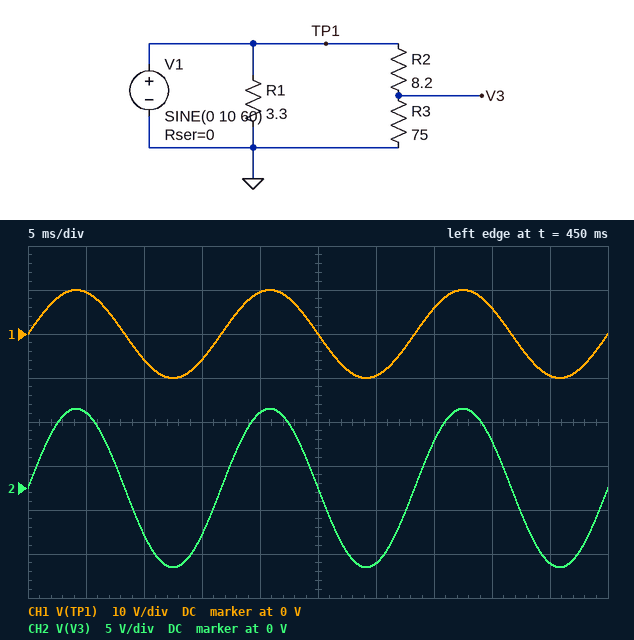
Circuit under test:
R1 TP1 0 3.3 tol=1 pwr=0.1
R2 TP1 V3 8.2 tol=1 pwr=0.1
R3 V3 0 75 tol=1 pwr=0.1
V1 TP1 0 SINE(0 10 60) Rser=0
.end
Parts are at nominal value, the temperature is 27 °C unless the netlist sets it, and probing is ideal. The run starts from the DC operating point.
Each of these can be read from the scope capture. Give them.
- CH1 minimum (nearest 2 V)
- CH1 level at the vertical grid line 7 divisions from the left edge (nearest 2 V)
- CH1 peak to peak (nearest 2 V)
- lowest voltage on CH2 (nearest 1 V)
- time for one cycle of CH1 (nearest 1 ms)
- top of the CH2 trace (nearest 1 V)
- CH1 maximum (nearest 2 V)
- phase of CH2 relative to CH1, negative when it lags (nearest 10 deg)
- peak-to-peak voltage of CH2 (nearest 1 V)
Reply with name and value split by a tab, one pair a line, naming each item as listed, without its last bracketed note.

CH1 minimum	-10 V
CH1 level at the vertical grid line 7 divisions from the left edge	6 V
CH1 peak to peak	20 V
lowest voltage on CH2	-9 V
time for one cycle of CH1	17 ms
top of the CH2 trace	9 V
CH1 maximum	10 V
phase of CH2 relative to CH1, negative when it lags	0 deg
peak-to-peak voltage of CH2	18 V
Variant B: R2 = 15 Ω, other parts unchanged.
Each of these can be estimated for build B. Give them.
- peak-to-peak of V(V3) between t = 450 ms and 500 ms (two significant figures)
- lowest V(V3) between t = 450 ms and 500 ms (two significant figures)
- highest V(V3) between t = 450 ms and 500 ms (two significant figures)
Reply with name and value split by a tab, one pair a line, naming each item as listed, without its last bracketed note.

peak-to-peak of V(V3) between t = 450 ms and 500 ms	17 V
lowest V(V3) between t = 450 ms and 500 ms	-8.3 V
highest V(V3) between t = 450 ms and 500 ms	8.3 V
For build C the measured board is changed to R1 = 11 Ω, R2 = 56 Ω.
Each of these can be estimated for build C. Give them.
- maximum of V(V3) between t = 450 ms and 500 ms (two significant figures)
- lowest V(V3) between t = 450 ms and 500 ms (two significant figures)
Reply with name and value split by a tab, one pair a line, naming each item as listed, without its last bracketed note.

maximum of V(V3) between t = 450 ms and 500 ms	5.7 V
lowest V(V3) between t = 450 ms and 500 ms	-5.7 V
